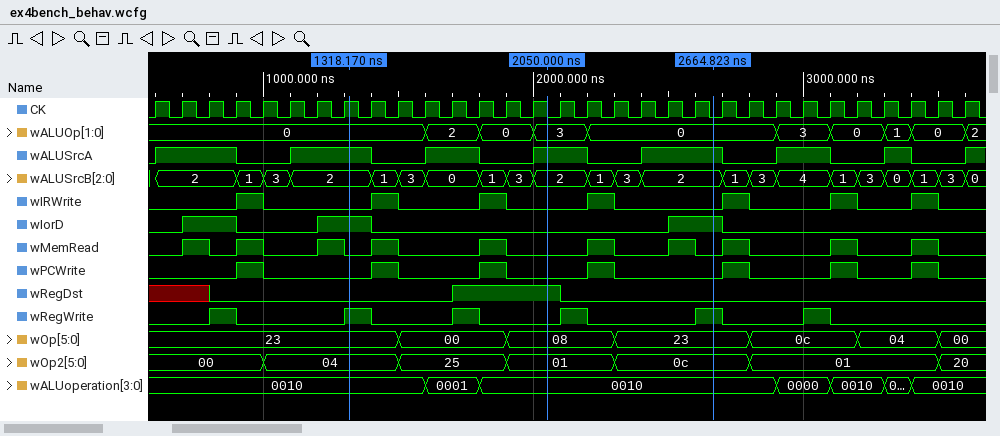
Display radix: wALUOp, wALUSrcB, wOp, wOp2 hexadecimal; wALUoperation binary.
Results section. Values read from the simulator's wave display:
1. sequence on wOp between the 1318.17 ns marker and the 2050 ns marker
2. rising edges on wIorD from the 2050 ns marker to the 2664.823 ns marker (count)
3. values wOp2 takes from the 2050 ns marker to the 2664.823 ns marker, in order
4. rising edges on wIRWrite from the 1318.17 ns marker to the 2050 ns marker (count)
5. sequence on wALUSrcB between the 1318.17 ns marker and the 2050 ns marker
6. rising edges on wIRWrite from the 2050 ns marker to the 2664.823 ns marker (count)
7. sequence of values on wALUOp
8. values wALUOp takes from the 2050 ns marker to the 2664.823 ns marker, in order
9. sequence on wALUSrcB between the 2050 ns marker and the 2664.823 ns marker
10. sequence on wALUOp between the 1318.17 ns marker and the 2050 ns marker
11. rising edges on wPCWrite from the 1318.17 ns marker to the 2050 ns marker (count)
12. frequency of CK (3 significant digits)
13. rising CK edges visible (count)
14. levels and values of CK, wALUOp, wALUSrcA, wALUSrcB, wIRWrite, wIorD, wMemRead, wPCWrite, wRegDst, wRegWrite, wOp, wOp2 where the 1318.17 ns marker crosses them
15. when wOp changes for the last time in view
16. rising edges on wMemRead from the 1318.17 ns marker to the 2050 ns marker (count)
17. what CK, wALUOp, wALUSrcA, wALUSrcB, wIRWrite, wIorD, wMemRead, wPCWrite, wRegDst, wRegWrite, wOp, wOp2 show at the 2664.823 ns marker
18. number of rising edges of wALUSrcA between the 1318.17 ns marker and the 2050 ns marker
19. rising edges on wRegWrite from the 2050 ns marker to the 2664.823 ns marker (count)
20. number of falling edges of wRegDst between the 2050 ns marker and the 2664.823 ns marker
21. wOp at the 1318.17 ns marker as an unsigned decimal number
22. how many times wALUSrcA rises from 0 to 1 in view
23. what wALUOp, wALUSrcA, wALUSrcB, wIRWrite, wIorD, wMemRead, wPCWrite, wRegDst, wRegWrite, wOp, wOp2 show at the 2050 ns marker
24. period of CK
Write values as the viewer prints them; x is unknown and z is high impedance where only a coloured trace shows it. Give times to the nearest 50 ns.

23, 00, 08
1
01, 0c
2
2, 1, 3, 0, 1, 3, 2
1
0, 2, 0, 3, 0, 3, 0, 1, 0, 2
3, 0
2, 1, 3, 2
0, 2, 0, 3
2
10.0 MHz
31
CK=1, wALUOp=0, wALUSrcA=1, wALUSrcB=2, wIRWrite=0, wIorD=1, wMemRead=0, wPCWrite=0, wRegDst=0, wRegWrite=1, wOp=23, wOp2=04
3500 ns
2
CK=0, wALUOp=0, wALUSrcA=1, wALUSrcB=2, wIRWrite=0, wIorD=1, wMemRead=0, wPCWrite=0, wRegDst=0, wRegWrite=1, wOp=23, wOp2=0c
2
2
1
35
8
wALUOp=3, wALUSrcA=1, wALUSrcB=2, wIRWrite=0, wIorD=0, wMemRead=0, wPCWrite=0, wRegDst=1, wRegWrite=0, wOp=08, wOp2=01
100 ns
